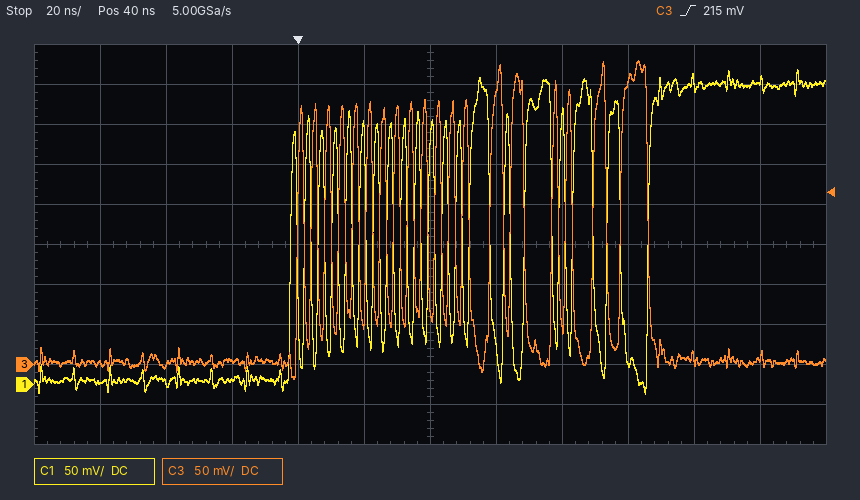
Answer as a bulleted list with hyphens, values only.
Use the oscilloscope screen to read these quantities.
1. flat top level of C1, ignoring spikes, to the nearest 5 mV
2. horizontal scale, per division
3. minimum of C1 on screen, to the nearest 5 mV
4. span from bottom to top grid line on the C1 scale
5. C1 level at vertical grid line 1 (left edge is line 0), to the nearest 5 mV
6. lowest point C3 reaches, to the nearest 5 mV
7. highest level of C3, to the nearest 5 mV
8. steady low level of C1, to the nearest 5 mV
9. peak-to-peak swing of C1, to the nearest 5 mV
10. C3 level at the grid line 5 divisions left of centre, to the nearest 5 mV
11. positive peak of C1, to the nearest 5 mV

- 375 mV
- 20 ns
- -10 mV
- 500 mV
- 5 mV
- -20 mV
- 380 mV
- 5 mV
- 405 mV
- 0 mV
- 395 mV
